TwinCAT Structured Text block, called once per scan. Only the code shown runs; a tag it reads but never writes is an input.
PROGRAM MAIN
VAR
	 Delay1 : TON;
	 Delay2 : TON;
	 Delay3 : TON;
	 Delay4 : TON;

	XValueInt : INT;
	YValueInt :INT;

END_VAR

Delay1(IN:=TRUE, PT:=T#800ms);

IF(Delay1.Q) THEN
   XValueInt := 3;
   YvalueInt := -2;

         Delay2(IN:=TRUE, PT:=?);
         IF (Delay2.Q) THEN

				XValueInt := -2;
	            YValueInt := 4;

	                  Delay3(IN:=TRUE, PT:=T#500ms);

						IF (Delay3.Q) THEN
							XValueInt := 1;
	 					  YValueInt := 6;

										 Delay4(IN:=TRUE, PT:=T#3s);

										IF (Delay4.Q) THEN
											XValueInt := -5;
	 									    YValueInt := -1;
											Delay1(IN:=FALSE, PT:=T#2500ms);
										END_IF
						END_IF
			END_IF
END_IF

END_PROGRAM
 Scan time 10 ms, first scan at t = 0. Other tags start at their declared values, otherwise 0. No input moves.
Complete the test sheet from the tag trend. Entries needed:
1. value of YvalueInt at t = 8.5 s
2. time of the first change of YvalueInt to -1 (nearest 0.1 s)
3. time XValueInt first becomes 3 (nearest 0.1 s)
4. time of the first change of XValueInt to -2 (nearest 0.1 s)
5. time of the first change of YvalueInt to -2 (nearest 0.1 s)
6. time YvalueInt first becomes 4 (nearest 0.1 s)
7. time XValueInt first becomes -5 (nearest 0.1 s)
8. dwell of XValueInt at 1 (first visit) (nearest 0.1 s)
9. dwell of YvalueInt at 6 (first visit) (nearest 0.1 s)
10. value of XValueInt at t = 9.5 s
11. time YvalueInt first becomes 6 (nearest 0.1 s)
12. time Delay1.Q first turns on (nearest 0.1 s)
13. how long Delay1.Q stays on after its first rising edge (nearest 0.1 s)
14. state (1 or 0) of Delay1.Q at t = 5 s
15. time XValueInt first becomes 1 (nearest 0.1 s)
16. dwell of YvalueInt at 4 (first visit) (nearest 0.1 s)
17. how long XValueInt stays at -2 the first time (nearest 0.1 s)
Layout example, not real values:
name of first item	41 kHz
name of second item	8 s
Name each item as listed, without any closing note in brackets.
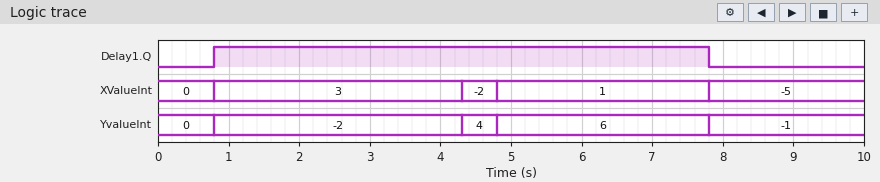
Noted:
value of YvalueInt at t = 8.5 s	-1
time of the first change of YvalueInt to -1	7.8 s
time XValueInt first becomes 3	0.8 s
time of the first change of XValueInt to -2	4.3 s
time of the first change of YvalueInt to -2	0.8 s
time YvalueInt first becomes 4	4.3 s
time XValueInt first becomes -5	7.8 s
dwell of XValueInt at 1 (first visit)	3.0 s
dwell of YvalueInt at 6 (first visit)	3.0 s
value of XValueInt at t = 9.5 s	-5
time YvalueInt first becomes 6	4.8 s
time Delay1.Q first turns on	0.8 s
how long Delay1.Q stays on after its first rising edge	7.0 s
state (1 or 0) of Delay1.Q at t = 5 s	1
time XValueInt first becomes 1	4.8 s
dwell of YvalueInt at 4 (first visit)	0.5 s
how long XValueInt stays at -2 the first time	0.5 s
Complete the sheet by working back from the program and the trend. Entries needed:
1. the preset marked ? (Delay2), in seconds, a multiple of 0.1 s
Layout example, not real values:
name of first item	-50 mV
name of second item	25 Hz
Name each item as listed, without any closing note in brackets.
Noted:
the preset marked ? (Delay2), in seconds, a multiple of 0.1 s	3.5 s
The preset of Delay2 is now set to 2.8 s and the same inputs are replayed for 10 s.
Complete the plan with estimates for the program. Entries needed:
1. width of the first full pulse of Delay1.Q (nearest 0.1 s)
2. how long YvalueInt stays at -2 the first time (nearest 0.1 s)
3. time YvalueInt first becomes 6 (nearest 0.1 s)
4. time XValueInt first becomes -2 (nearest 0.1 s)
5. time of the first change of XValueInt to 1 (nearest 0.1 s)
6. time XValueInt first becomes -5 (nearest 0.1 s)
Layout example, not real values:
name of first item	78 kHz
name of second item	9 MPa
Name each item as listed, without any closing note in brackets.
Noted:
width of the first full pulse of Delay1.Q	6.3 s
how long YvalueInt stays at -2 the first time	2.8 s
time YvalueInt first becomes 6	4.1 s
time XValueInt first becomes -2	3.6 s
time of the first change of XValueInt to 1	4.1 s
time XValueInt first becomes -5	7.1 s
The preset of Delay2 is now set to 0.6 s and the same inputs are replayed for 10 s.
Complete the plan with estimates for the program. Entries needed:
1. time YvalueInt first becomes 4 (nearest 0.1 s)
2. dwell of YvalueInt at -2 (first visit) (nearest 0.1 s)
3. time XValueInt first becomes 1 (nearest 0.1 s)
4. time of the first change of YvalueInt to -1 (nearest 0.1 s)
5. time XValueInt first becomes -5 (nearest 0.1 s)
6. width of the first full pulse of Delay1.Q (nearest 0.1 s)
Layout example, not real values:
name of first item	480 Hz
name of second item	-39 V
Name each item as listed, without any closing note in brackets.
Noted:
time YvalueInt first becomes 4	1.4 s
dwell of YvalueInt at -2 (first visit)	0.6 s
time XValueInt first becomes 1	1.9 s
time of the first change of YvalueInt to -1	4.9 s
time XValueInt first becomes -5	4.9 s
width of the first full pulse of Delay1.Q	4.1 s
